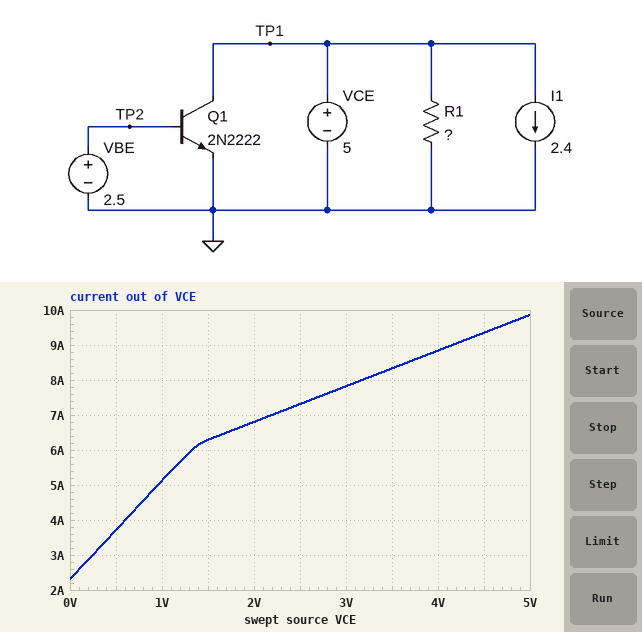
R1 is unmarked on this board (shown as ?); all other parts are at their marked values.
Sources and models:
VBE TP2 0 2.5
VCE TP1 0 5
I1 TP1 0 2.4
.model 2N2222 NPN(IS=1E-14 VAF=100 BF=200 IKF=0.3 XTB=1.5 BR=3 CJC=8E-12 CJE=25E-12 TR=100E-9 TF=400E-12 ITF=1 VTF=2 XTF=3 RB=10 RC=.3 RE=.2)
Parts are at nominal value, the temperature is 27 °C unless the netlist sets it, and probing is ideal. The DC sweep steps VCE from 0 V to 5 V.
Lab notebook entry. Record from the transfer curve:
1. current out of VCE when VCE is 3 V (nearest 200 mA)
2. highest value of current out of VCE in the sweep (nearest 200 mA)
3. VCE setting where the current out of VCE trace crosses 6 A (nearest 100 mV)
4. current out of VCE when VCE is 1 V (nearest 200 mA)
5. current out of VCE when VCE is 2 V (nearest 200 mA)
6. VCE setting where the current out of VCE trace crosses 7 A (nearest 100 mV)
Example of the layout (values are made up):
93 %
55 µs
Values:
7.8 A
9.8 A
1.3 V
5.2 A
6.8 A
2.2 V
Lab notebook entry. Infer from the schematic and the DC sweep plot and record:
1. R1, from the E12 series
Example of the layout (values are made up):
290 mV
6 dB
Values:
1 Ω
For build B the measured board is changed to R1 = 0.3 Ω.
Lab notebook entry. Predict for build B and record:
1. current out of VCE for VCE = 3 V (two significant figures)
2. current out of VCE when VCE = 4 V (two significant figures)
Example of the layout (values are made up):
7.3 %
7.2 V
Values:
15 A
18 A
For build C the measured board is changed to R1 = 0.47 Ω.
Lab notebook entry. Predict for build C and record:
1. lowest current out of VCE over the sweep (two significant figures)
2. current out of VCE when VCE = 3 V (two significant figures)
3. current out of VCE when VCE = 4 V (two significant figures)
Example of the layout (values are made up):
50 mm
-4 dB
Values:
2.3 A
11 A
13 A
